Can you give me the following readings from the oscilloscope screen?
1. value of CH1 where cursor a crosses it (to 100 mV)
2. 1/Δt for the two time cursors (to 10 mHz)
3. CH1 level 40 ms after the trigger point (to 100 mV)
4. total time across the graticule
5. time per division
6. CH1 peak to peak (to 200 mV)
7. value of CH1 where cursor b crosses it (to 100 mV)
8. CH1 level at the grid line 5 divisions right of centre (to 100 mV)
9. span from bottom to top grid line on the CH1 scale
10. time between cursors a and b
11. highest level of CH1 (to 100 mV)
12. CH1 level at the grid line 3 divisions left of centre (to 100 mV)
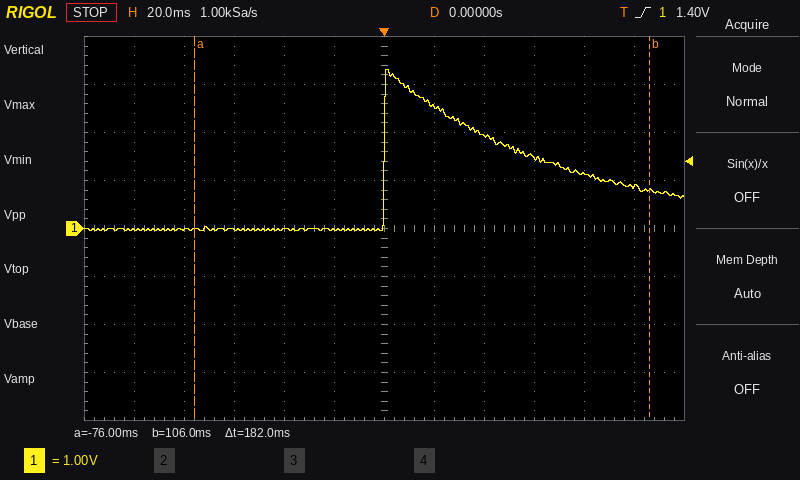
0.0 V
5.49 Hz
1.9 V
240 ms
20 ms
3.4 V
800 mV
900 mV
8 V
182 ms
3.3 V
0.0 V
